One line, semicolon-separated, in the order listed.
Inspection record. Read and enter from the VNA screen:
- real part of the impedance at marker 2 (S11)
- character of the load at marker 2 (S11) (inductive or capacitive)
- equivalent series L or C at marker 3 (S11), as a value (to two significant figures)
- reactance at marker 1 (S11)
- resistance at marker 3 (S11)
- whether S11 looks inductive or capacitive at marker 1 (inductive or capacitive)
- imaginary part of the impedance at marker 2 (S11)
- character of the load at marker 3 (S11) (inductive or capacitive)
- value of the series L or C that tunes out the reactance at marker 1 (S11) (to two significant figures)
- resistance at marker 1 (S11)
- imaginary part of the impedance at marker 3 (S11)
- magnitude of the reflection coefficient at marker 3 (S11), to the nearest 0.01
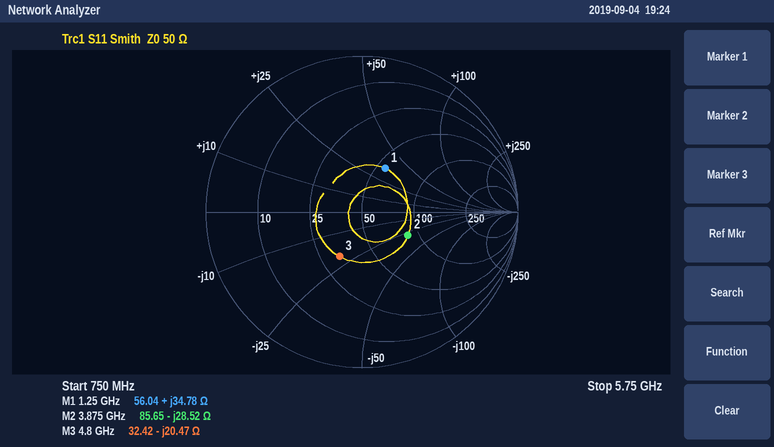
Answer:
85.65 Ω; capacitive; 1.6 pF; +34.78 Ω; 32.42 Ω; inductive; -28.52 Ω; capacitive; 3.7 pF; 56.04 Ω; -20.47 Ω; 0.32
